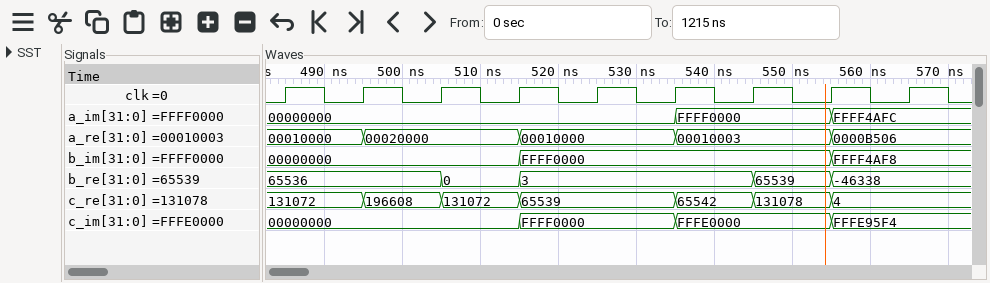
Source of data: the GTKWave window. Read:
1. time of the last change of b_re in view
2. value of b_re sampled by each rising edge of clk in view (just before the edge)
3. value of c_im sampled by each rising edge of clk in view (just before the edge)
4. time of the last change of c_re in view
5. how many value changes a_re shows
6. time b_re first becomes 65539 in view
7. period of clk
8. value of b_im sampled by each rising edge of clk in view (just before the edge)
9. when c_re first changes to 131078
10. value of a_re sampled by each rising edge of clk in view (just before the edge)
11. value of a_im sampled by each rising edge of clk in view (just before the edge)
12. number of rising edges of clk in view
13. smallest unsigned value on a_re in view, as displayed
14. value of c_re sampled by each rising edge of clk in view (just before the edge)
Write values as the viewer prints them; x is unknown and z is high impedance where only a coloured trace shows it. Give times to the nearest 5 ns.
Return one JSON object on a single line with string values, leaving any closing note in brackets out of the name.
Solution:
{"time of the last change of b_re in view": "555 ns", "value of b_re sampled by each rising edge of clk in view": "65536, 65536, 65536, 0, 3, 3, 3, 65539, -46338", "value of c_im sampled by each rising edge of clk in view": "00000000, 00000000, 00000000, 00000000, FFFF0000, FFFF0000, FFFE0000, FFFE0000, FFFE95F4", "time of the last change of c_re in view": "555 ns", "how many value changes a_re shows": "4", "time b_re first becomes 65539 in view": "545 ns", "period of clk": "10 ns", "value of b_im sampled by each rising edge of clk in view": "00000000, 00000000, 00000000, 00000000, FFFF0000, FFFF0000, FFFF0000, FFFF0000, FFFF4AF8", "when c_re first changes to 131078": "545 ns", "value of a_re sampled by each rising edge of clk in view": "00010000, 00010000, 00020000, 00020000, 00010000, 00010000, 00010003, 00010003, 0000B506", "value of a_im sampled by each rising edge of clk in view": "00000000, 00000000, 00000000, 00000000, 00000000, 00000000, FFFF0000, FFFF0000, FFFF4AFC", "number of rising edges of clk in view": "9", "smallest unsigned value on a_re in view, as displayed": "0000B506", "value of c_re sampled by each rising edge of clk in view": "131072, 131072, 196608, 131072, 65539, 65539, 65542, 131078, 4"}
